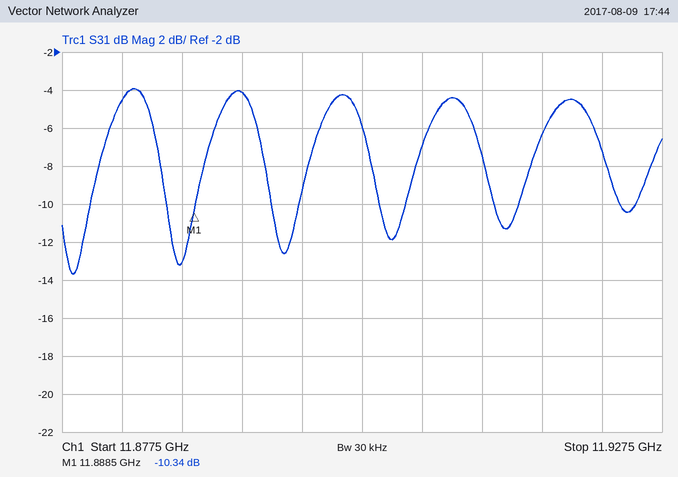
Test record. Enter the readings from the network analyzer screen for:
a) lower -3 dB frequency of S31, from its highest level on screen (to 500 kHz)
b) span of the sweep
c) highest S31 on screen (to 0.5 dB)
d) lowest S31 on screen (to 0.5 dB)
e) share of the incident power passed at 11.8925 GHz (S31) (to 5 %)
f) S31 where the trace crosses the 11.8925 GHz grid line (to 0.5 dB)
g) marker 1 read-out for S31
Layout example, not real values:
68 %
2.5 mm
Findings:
11.8810 GHz
50 MHz
-4.0 dB
-13.5 dB
40 %
-4.0 dB
-10.34 dB
